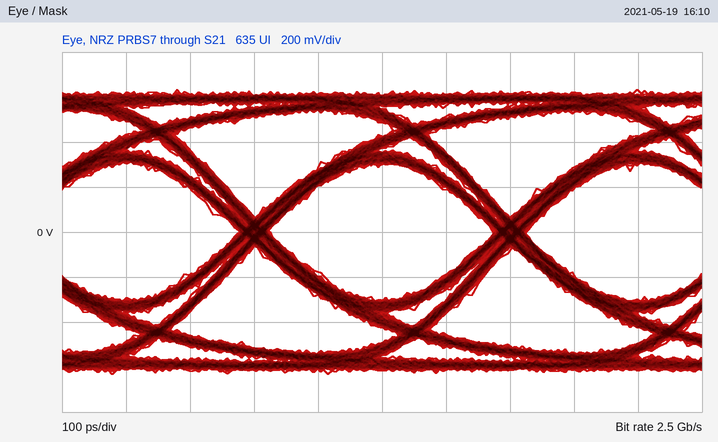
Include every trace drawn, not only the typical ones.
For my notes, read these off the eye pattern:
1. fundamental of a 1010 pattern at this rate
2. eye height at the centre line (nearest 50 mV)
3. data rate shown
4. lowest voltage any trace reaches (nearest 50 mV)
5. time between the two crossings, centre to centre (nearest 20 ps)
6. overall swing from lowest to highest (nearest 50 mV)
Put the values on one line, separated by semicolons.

1.25 GHz; 600 mV; 2.5 Gb/s; -650 mV; 400 ps; 1.25 V
